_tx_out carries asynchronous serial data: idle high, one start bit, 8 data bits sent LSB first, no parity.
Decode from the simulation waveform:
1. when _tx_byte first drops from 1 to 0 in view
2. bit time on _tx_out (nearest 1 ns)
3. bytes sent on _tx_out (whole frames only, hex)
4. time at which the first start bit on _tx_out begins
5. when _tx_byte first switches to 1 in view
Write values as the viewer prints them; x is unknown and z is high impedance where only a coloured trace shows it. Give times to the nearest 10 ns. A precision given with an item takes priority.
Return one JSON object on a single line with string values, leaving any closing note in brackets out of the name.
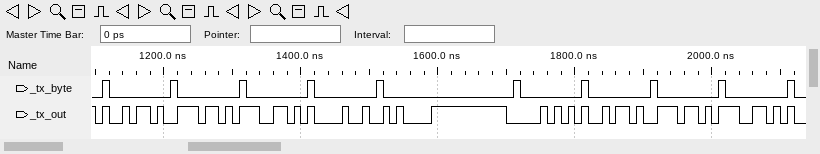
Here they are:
{"when _tx_byte first drops from 1 to 0 in view": "1120 ns", "bit time on _tx_out": "10 ns", "bytes sent on _tx_out": "69, 6E, 67, 21, 0A, 50, 69, 6E, 67", "time at which the first start bit on _tx_out begins": "1100 ns", "when _tx_byte first switches to 1 in view": "1110 ns"}
